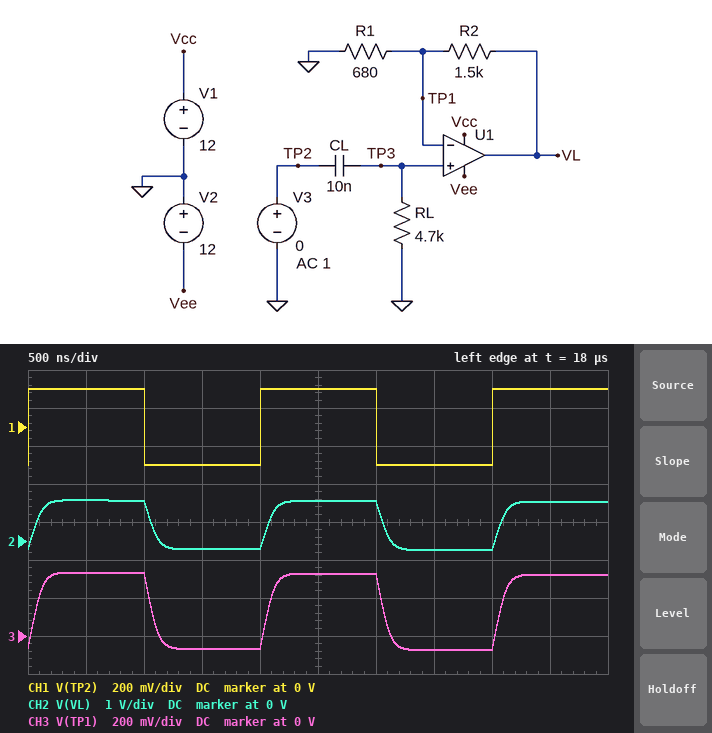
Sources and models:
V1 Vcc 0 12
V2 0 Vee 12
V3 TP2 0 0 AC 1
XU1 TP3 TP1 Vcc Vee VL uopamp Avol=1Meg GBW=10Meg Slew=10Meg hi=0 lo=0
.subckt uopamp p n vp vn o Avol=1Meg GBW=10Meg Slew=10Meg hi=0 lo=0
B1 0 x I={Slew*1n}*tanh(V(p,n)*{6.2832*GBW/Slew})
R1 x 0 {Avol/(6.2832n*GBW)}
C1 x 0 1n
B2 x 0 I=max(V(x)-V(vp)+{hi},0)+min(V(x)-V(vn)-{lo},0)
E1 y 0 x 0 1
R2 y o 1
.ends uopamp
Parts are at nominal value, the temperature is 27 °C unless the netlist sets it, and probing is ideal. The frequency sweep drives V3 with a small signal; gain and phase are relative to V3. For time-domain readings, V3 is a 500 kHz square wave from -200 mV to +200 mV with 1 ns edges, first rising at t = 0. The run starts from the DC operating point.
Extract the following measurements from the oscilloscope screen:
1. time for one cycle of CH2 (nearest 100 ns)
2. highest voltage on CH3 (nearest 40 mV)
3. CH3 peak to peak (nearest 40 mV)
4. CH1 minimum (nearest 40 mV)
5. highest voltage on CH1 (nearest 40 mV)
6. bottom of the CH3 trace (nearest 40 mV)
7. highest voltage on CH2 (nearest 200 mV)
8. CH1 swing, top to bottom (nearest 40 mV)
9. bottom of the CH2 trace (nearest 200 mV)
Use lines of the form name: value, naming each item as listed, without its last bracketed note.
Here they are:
time for one cycle of CH2: 2.0 µs
highest voltage on CH3: 320 mV
CH3 peak to peak: 400 mV
CH1 minimum: -200 mV
highest voltage on CH1: 200 mV
bottom of the CH3 trace: -80 mV
highest voltage on CH2: 1.0 V
CH1 swing, top to bottom: 400 mV
bottom of the CH2 trace: -200 mV
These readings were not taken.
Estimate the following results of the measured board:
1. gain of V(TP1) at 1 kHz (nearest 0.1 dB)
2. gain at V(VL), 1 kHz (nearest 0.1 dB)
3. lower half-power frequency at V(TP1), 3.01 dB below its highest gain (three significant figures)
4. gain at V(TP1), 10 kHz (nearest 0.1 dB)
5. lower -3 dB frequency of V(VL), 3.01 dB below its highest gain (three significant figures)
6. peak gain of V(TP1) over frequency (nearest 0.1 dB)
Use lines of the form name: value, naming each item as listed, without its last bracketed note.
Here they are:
gain of V(TP1) at 1 kHz: -11.0 dB
gain at V(VL), 1 kHz: -0.8 dB
lower half-power frequency at V(TP1), 3.01 dB below its highest gain: 3.38 kHz
gain at V(TP1), 10 kHz: -0.5 dB
lower -3 dB frequency of V(VL), 3.01 dB below its highest gain: 3.38 kHz
peak gain of V(TP1) over frequency: 0 dB
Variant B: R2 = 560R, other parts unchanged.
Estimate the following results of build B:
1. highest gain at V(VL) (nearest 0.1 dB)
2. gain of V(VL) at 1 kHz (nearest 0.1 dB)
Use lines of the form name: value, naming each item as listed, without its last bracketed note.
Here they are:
highest gain at V(VL): 5.2 dB
gain of V(VL) at 1 kHz: -5.7 dB
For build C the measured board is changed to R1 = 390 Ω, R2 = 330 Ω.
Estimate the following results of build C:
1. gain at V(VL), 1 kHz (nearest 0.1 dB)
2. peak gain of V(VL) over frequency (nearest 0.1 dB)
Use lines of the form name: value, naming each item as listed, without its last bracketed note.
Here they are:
gain at V(VL), 1 kHz: -5.6 dB
peak gain of V(VL) over frequency: 5.3 dB
